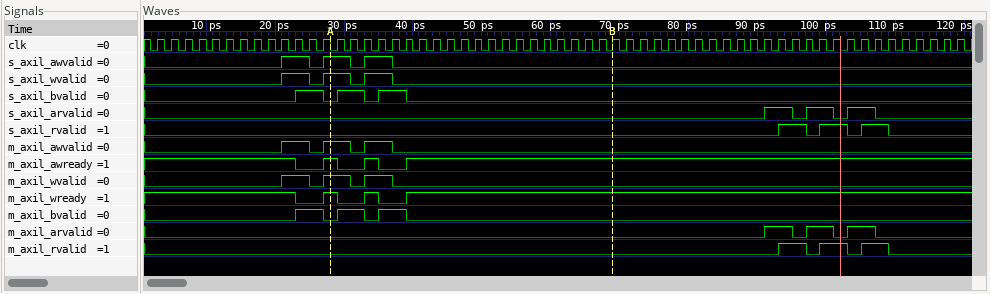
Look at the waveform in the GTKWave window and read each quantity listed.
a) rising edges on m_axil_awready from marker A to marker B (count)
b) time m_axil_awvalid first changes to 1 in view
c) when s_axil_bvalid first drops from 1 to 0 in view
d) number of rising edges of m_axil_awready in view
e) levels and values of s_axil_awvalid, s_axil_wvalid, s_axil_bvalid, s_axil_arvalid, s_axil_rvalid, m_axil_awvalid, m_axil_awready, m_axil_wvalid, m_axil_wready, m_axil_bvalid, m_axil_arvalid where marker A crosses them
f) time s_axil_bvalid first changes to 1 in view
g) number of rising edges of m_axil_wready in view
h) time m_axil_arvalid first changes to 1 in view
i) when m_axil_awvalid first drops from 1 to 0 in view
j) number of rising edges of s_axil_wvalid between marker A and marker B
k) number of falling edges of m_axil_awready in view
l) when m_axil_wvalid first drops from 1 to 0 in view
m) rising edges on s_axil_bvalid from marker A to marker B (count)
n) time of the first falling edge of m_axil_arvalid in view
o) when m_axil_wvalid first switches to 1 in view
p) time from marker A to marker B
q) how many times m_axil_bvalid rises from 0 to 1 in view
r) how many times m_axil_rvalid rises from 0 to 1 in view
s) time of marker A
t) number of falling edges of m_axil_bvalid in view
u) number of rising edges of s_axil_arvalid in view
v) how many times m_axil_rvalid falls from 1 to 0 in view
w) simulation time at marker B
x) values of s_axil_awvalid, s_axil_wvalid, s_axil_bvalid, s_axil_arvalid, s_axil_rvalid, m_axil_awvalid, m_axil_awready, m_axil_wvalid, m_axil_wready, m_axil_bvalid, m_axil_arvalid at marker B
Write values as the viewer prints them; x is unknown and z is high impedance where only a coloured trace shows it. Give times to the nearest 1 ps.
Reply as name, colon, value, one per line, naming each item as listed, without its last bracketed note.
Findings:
rising edges on m_axil_awready from marker A to marker B: 2
time m_axil_awvalid first changes to 1 in view: 21 ps
when s_axil_bvalid first drops from 1 to 0 in view: 27 ps
number of rising edges of m_axil_awready in view: 3
levels and values of s_axil_awvalid, s_axil_wvalid, s_axil_bvalid, s_axil_arvalid, s_axil_rvalid, m_axil_awvalid, m_axil_awready, m_axil_wvalid, m_axil_wready, m_axil_bvalid, m_axil_arvalid where marker A crosses them: s_axil_awvalid=1, s_axil_wvalid=1, s_axil_bvalid=0, s_axil_arvalid=0, s_axil_rvalid=0, m_axil_awvalid=1, m_axil_awready=1, m_axil_wvalid=1, m_axil_wready=1, m_axil_bvalid=0, m_axil_arvalid=0
time s_axil_bvalid first changes to 1 in view: 23 ps
number of rising edges of m_axil_wready in view: 3
time m_axil_arvalid first changes to 1 in view: 91 ps
when m_axil_awvalid first drops from 1 to 0 in view: 25 ps
number of rising edges of s_axil_wvalid between marker A and marker B: 1
number of falling edges of m_axil_awready in view: 3
when m_axil_wvalid first drops from 1 to 0 in view: 25 ps
rising edges on s_axil_bvalid from marker A to marker B: 2
time of the first falling edge of m_axil_arvalid in view: 95 ps
when m_axil_wvalid first switches to 1 in view: 21 ps
time from marker A to marker B: 41 ps
how many times m_axil_bvalid rises from 0 to 1 in view: 3
how many times m_axil_rvalid rises from 0 to 1 in view: 3
time of marker A: 28 ps
number of falling edges of m_axil_bvalid in view: 3
number of rising edges of s_axil_arvalid in view: 3
how many times m_axil_rvalid falls from 1 to 0 in view: 3
simulation time at marker B: 69 ps
values of s_axil_awvalid, s_axil_wvalid, s_axil_bvalid, s_axil_arvalid, s_axil_rvalid, m_axil_awvalid, m_axil_awready, m_axil_wvalid, m_axil_wready, m_axil_bvalid, m_axil_arvalid at marker B: s_axil_awvalid=0, s_axil_wvalid=0, s_axil_bvalid=0, s_axil_arvalid=0, s_axil_rvalid=0, m_axil_awvalid=0, m_axil_awready=1, m_axil_wvalid=0, m_axil_wready=1, m_axil_bvalid=0, m_axil_arvalid=0
